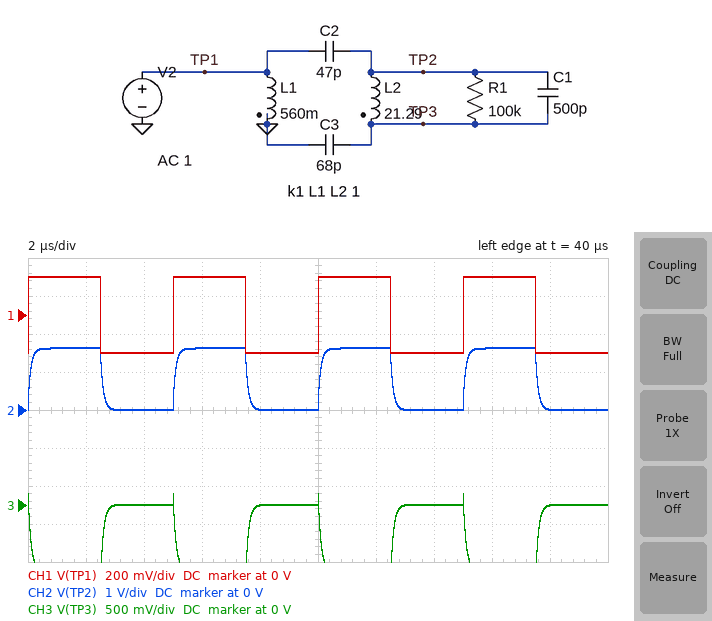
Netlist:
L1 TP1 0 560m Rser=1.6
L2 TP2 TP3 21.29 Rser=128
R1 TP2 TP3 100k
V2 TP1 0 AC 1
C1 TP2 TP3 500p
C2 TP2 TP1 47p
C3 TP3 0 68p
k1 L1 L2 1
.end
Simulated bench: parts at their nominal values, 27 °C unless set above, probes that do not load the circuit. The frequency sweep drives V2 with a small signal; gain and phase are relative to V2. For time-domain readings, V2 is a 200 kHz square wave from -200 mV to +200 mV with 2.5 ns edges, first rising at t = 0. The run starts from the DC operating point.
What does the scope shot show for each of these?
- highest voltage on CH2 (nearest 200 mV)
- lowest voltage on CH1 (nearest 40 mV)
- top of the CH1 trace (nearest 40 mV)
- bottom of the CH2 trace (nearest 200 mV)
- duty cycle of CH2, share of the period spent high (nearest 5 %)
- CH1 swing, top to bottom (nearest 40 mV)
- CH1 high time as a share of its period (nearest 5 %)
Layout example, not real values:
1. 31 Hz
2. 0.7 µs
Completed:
1. 1.6 V
2. -200 mV
3. 200 mV
4. 0 V
5. 50 %
6. 400 mV
7. 50 %
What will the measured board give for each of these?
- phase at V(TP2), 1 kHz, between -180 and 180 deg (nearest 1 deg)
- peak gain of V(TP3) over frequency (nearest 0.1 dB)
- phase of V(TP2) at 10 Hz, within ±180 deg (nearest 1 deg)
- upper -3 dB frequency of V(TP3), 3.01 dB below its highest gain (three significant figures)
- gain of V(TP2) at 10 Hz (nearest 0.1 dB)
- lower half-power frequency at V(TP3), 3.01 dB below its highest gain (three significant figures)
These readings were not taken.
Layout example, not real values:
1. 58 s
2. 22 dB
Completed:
1. 0 deg
2. 6.5 dB
3. 2 deg
4. 1.66 MHz
5. 12.1 dB
6. 437 mHz
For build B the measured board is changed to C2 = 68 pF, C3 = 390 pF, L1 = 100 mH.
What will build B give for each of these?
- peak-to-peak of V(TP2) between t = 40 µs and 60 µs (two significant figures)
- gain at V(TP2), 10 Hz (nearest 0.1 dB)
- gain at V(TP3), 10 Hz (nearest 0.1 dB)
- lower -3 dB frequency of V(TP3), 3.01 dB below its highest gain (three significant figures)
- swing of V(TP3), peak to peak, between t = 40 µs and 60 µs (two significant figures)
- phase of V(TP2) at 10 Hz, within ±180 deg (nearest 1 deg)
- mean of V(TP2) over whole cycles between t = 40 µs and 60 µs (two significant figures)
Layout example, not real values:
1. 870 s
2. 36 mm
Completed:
1. 5.0 V
2. 21.7 dB
3. 5.8 dB
4. 2.52 Hz
5. 900 mV
6. 14 deg
7. 2.5 V
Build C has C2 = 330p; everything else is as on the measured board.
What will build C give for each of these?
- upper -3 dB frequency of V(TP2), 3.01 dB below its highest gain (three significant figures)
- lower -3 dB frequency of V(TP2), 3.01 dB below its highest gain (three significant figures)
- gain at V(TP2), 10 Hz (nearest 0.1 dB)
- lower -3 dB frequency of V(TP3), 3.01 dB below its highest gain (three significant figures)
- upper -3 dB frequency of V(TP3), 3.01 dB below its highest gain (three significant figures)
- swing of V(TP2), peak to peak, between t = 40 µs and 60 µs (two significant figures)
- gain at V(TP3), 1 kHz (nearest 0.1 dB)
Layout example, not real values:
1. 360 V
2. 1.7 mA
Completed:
1. 1.97 MHz
2. 355 mHz
3. 5.5 dB
4. 437 mHz
5. 1.57 MHz
6. 750 mV
7. 12.6 dB
